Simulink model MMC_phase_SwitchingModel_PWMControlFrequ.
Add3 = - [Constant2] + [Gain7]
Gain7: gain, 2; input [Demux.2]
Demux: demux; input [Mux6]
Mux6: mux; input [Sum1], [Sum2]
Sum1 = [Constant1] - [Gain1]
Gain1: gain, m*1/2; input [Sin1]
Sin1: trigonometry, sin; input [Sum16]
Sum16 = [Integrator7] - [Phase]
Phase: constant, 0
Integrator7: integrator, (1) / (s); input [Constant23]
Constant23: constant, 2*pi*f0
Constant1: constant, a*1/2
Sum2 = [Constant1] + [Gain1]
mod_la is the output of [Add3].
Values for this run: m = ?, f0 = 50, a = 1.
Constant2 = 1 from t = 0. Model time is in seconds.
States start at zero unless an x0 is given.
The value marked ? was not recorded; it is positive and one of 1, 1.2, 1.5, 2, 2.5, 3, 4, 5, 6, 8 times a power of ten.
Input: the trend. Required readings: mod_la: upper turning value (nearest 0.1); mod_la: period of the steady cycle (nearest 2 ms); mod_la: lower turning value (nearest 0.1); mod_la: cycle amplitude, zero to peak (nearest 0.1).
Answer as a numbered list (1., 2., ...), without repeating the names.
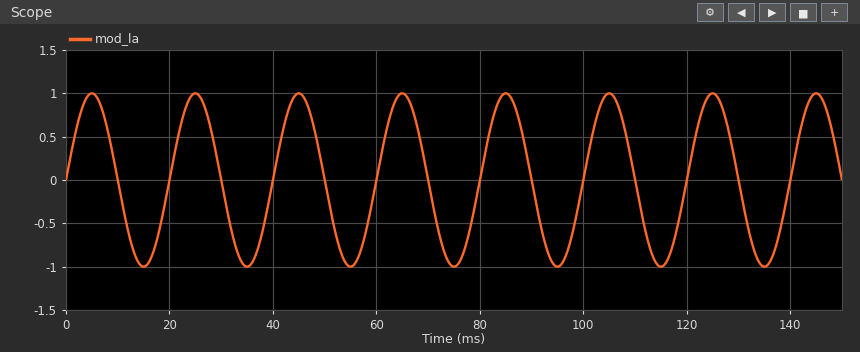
1. 1.0
2. 20 ms
3. -1.0
4. 1.0
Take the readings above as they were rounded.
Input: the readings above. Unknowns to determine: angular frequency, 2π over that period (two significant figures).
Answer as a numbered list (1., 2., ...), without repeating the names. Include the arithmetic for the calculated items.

1. 2π / 20 = 0.31 rad/ms
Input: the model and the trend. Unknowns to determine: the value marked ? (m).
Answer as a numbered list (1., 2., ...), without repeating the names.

1. 1
